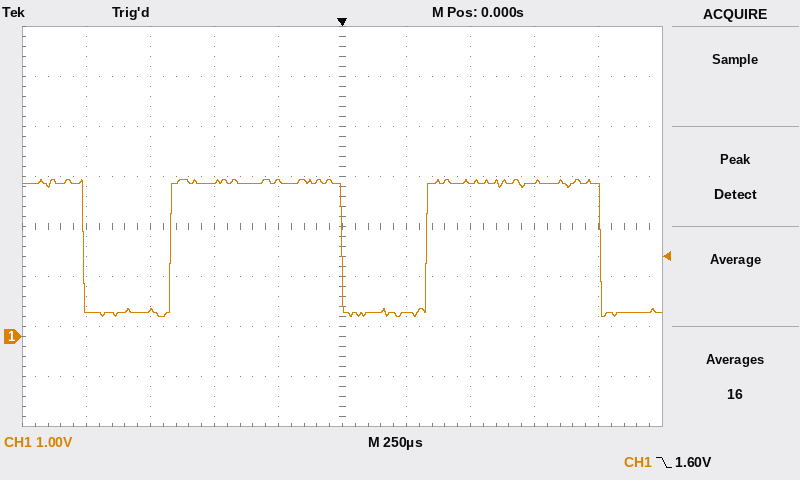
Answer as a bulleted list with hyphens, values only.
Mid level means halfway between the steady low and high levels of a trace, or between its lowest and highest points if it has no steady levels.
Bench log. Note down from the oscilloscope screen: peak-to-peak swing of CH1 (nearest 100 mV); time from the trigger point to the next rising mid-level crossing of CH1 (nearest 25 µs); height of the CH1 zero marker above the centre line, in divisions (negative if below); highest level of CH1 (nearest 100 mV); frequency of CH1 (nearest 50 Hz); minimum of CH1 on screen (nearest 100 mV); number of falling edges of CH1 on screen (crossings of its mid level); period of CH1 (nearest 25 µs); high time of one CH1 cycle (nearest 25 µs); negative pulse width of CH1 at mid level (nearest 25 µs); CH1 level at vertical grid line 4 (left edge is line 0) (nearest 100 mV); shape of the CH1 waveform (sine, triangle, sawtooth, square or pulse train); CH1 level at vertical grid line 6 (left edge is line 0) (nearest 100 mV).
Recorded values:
- 2.7 V
- 325 µs
- -2.2 div
- 3.1 V
- 1.00 kHz
- 400 mV
- 3
- 1.000 ms
- 675 µs
- 325 µs
- 3.1 V
- pulse train
- 500 mV
